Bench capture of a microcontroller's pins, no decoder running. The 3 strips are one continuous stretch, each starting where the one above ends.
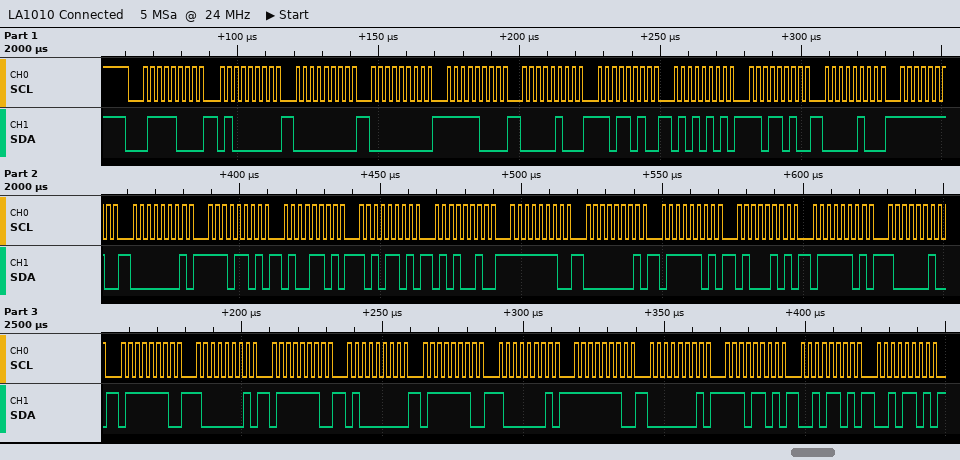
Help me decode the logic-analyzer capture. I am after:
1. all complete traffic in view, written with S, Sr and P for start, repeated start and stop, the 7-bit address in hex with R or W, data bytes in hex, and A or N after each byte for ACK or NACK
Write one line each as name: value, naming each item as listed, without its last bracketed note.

all complete traffic in view, written with S, Sr and P for start, repeated start and stop, the 7-bit address in hex with R or W, data bytes in hex, and A or N after each byte for ACK or NACK: S 3CW A 40 A 00 A 00 A F8 A 04 A DA A 55 A DA A 04 A FE A 01 A ED A 4D A AD A 52 A FE A 01 A 7D A 45 A 7D A 82 A 7E A 81 A 7E A 40 A 7E A 81 A FE A 01 A ED A 2D A 2D A
